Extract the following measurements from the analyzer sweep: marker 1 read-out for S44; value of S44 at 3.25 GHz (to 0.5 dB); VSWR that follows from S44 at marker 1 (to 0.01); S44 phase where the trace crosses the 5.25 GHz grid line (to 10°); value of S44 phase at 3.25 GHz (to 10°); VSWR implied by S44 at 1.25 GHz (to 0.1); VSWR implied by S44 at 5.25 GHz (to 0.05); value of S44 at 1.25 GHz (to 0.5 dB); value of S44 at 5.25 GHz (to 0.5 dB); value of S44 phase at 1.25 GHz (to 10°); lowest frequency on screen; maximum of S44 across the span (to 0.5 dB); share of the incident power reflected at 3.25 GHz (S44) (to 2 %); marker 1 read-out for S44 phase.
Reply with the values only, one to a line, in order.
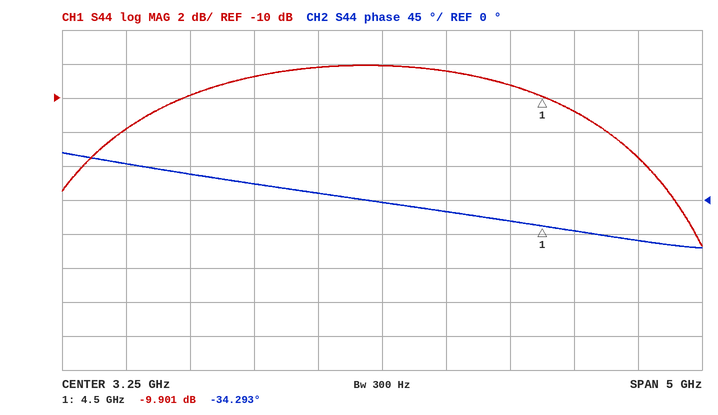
-9.901 dB
-8.0 dB
1.94
-50°
0°
1.7
1.55
-12.0 dB
-13.5 dB
50°
750 MHz
-8.0 dB
16 %
-34.293°
